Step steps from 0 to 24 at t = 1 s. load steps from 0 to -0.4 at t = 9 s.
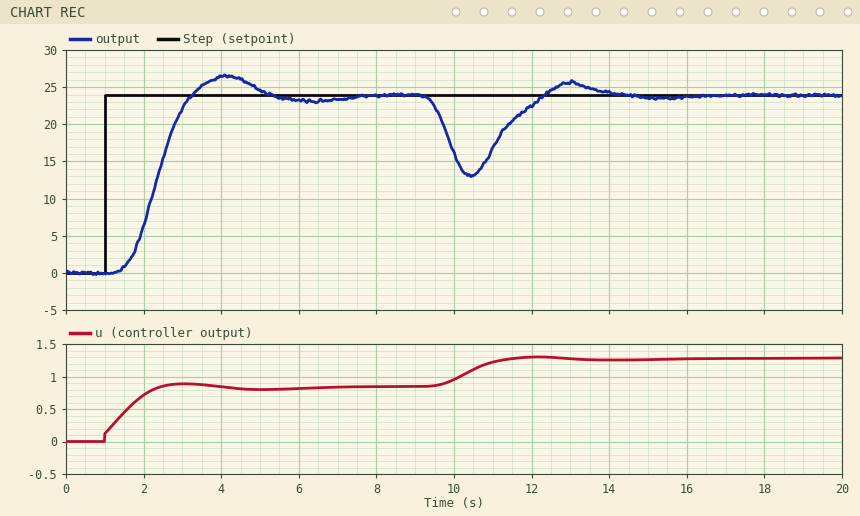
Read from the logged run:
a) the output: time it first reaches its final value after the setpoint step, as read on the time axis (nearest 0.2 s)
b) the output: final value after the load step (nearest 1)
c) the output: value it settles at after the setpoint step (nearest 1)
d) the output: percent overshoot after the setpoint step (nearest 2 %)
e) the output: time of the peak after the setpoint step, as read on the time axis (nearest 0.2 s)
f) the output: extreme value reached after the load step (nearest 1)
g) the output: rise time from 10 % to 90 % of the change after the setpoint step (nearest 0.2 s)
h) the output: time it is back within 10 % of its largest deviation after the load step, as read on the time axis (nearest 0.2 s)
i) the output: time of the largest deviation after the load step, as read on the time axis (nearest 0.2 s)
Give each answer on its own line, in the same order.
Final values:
3.2 s
24
24
10 %
4.2 s
13
1.2 s
13.4 s
10.4 s
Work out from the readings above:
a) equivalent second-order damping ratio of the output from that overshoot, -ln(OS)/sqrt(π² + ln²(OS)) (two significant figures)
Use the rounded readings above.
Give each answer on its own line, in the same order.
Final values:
0.59
